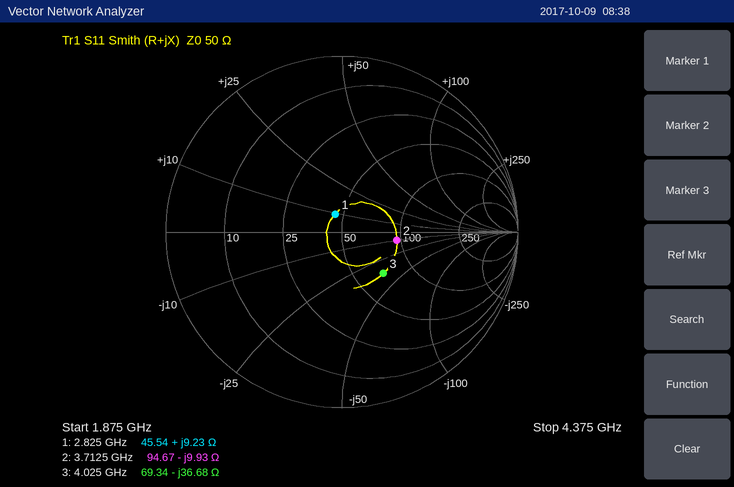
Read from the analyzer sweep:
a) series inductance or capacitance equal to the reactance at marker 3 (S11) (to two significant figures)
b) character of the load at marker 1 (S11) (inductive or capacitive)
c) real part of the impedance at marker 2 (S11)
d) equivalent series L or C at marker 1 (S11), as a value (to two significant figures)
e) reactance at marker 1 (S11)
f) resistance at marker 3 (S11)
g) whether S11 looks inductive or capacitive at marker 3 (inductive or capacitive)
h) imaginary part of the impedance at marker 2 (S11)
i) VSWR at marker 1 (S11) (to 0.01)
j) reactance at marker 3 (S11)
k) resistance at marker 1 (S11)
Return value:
1.1 pF
inductive
94.67 Ω
520 pH
+9.23 Ω
69.34 Ω
capacitive
-9.93 Ω
1.24
-36.68 Ω
45.54 Ω
